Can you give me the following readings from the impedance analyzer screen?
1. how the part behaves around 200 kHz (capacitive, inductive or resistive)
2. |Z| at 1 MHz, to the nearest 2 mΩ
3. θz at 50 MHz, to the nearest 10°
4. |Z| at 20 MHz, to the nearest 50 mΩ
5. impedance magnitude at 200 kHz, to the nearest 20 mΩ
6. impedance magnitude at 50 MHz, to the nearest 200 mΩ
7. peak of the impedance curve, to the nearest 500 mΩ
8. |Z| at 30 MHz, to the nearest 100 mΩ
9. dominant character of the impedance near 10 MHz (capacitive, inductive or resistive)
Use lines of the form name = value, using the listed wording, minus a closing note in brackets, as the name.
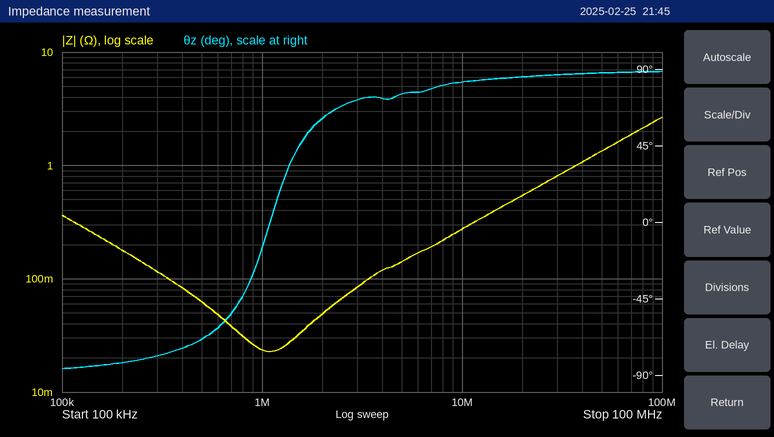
how the part behaves around 200 kHz = capacitive
|Z| at 1 MHz, to the nearest 2 mΩ = 24 mΩ
θz at 50 MHz, to the nearest 10° = 90°
|Z| at 20 MHz, to the nearest 50 mΩ = 550 mΩ
impedance magnitude at 200 kHz, to the nearest 20 mΩ = 180 mΩ
impedance magnitude at 50 MHz, to the nearest 200 mΩ = 1.4 Ω
peak of the impedance curve, to the nearest 500 mΩ = 2.5 Ω
|Z| at 30 MHz, to the nearest 100 mΩ = 800 mΩ
dominant character of the impedance near 10 MHz = inductive
